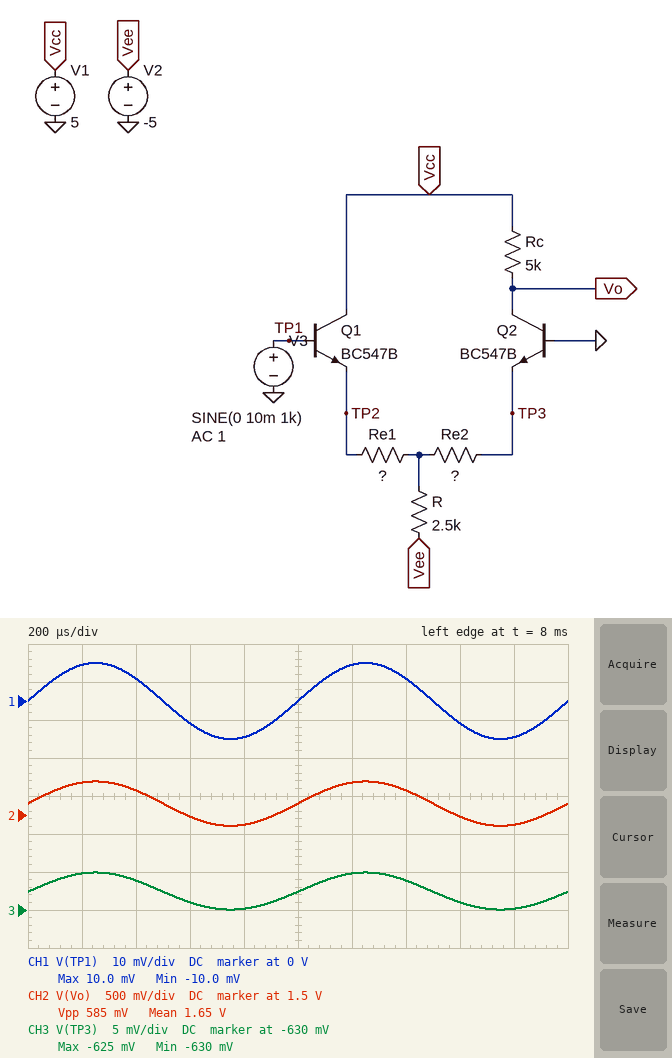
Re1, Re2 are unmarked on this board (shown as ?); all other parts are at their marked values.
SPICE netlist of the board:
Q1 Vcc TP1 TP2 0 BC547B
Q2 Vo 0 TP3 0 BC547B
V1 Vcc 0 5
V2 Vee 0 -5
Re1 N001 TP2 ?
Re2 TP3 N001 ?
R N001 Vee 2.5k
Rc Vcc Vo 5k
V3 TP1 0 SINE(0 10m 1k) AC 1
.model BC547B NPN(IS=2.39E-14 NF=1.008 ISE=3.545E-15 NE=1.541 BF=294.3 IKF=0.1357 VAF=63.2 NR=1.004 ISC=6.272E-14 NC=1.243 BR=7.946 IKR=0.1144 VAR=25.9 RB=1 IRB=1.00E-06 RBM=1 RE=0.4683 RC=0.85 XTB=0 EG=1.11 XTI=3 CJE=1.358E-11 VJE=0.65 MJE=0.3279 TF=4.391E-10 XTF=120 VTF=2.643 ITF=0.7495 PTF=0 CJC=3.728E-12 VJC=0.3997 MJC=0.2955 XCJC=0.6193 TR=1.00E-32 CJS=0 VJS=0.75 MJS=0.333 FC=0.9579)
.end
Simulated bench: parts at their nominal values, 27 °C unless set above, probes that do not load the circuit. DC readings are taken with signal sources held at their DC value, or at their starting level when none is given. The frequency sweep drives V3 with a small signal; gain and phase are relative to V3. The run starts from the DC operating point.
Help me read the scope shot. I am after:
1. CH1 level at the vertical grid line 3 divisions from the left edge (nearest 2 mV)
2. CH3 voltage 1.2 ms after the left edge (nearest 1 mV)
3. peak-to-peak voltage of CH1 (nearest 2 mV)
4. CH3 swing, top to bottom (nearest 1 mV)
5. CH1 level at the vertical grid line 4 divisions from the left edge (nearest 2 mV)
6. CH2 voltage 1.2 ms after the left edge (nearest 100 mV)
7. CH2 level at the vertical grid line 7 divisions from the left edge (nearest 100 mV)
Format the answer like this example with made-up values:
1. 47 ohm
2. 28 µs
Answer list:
1. -6 mV
2. -625 mV
3. 20 mV
4. 5 mV
5. -10 mV
6. 1.9 V
7. 1.8 V
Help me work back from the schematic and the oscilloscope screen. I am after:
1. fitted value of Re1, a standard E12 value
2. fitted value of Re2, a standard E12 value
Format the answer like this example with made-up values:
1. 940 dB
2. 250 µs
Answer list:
1. 33 Ω
2. 68 Ω
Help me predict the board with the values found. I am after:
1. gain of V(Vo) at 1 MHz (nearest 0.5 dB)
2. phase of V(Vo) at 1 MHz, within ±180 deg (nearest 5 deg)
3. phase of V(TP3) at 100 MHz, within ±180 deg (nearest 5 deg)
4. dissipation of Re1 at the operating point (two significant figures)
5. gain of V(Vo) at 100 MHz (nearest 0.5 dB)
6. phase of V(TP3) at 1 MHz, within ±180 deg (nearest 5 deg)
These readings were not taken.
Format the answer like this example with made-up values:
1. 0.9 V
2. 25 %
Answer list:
1. 29.5 dB
2. -5 deg
3. -35 deg
4. 37 µW
5. 10.0 dB
6. 0 deg
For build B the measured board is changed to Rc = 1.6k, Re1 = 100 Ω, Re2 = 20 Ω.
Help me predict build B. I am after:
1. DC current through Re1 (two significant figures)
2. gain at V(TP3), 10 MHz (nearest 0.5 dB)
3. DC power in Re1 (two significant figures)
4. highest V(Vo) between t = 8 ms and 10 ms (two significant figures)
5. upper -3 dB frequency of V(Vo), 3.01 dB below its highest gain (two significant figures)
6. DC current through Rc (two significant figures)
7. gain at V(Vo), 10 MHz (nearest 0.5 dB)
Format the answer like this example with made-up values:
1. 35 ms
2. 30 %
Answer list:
1. 500 µA
2. -19.0 dB
3. 25 µW
4. 3.1 V
5. 51 MHz
6. 1.2 mA
7. 18.0 dB
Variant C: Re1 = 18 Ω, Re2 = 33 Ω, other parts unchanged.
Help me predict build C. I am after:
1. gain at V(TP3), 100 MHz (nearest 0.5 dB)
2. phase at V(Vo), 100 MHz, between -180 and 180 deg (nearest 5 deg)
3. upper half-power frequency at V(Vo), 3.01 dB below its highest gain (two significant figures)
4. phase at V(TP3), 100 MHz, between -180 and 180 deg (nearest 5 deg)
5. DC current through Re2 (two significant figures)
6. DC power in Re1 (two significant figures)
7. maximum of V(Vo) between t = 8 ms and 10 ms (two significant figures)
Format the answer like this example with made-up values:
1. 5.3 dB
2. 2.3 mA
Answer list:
1. -11.5 dB
2. -110 deg
3. 13 MHz
4. -25 deg
5. 740 µA
6. 18 µW
7. 1.7 V
